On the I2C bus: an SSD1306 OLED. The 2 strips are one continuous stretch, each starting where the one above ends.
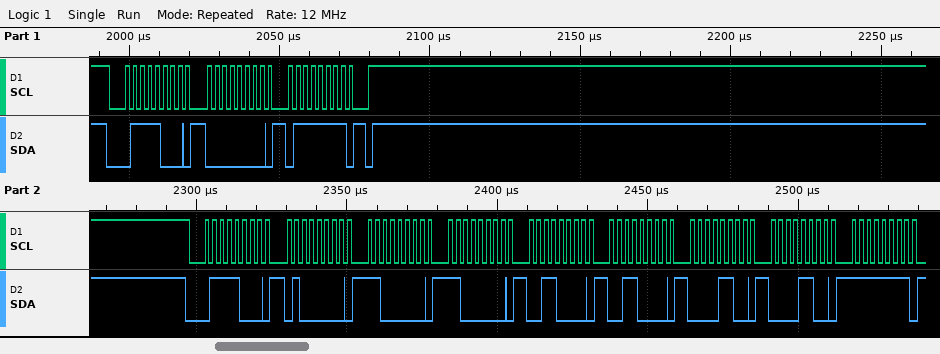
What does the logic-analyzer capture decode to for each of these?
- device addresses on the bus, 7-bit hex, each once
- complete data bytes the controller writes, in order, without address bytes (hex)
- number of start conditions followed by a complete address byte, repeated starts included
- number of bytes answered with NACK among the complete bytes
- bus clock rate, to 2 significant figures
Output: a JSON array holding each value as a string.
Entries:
["0x3C", "00 7F 40 C0 C0 30 30 0C 0C FF", "2", "0", "400 kHz"]
